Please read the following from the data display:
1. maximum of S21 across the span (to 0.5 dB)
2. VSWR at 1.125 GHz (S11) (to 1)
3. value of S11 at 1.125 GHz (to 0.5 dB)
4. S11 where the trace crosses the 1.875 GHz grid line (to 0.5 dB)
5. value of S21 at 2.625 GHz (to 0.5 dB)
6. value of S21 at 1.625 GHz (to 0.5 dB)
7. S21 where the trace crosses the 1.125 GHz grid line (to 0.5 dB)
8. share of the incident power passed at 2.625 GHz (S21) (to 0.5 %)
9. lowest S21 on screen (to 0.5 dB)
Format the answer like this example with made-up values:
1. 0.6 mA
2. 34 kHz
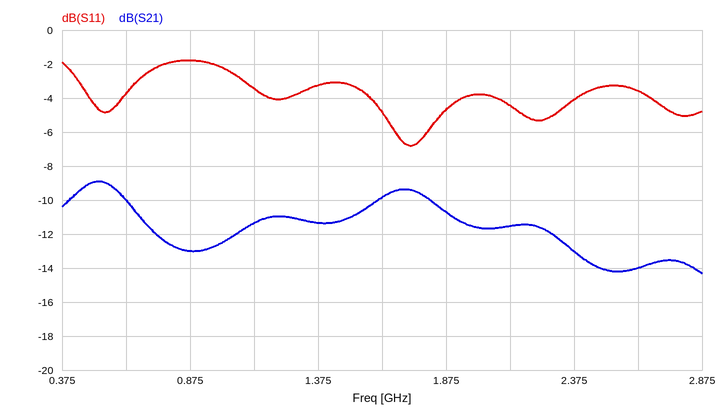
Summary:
1. -9.0 dB
2. 5
3. -3.5 dB
4. -4.5 dB
5. -14.0 dB
6. -10.0 dB
7. -11.5 dB
8. 4.0 %
9. -14.5 dB
